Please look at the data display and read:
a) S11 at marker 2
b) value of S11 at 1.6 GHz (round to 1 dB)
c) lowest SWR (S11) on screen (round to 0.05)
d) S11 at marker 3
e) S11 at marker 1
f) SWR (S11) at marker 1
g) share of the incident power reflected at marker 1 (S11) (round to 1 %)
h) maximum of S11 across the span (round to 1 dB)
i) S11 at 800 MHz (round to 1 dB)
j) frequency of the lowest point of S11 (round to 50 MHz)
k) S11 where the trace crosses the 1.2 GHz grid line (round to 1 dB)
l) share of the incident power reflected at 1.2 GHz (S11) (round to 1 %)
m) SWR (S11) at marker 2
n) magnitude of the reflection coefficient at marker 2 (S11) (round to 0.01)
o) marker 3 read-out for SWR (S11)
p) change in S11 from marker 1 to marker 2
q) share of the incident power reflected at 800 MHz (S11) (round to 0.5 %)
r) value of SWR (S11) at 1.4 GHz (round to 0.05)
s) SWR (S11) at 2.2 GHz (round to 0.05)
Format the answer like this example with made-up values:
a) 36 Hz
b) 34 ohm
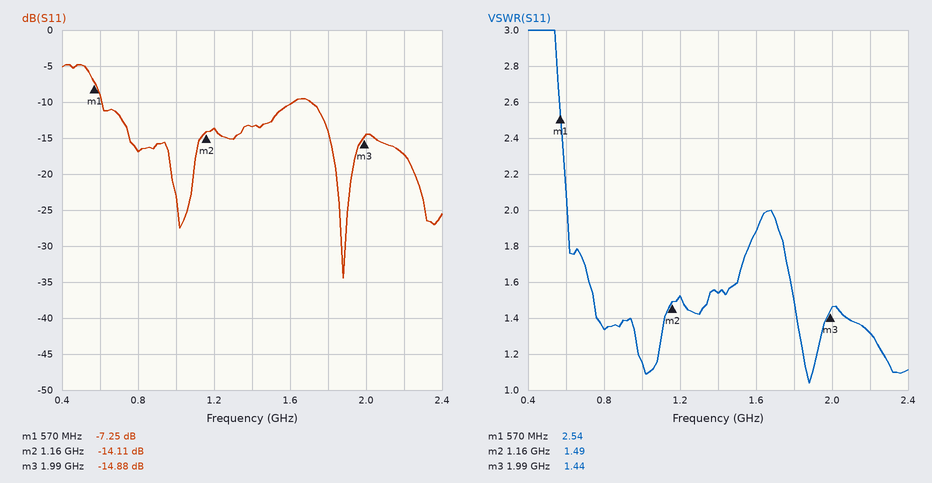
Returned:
a) -14.11 dB
b) -10 dB
c) 1.05
d) -14.88 dB
e) -7.25 dB
f) 2.54
g) 19 %
h) -5 dB
i) -17 dB
j) 1.90 GHz
k) -14 dB
l) 4 %
m) 1.49
n) 0.20
o) 1.44
p) -6.86 dB
q) 2.0 %
r) 1.55
s) 1.30
